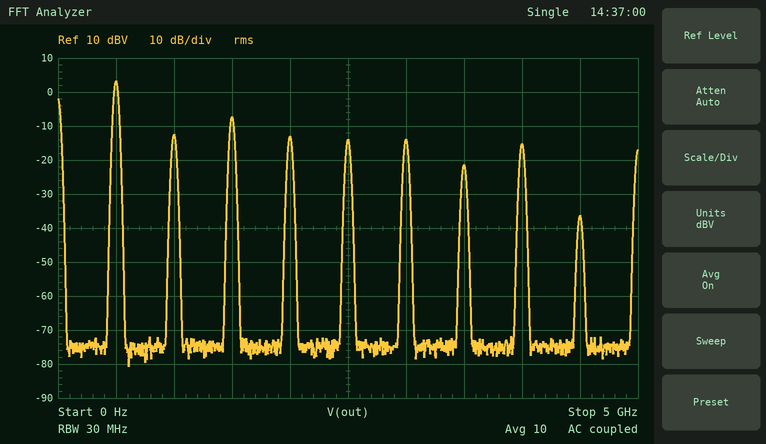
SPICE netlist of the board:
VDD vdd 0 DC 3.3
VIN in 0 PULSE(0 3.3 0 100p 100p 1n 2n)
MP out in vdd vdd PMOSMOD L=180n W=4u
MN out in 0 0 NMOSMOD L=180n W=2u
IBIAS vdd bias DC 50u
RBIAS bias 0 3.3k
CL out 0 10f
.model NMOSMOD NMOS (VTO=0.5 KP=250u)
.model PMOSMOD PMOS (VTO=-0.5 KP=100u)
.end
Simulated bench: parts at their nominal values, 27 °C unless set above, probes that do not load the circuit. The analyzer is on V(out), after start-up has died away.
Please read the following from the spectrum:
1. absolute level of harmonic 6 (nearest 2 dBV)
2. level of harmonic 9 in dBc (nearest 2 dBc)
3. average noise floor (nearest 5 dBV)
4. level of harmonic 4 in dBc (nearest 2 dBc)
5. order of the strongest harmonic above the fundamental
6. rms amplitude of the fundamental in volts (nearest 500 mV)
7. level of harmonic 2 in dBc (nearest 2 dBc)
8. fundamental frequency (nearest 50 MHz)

-14 dBV
-40 dBc
-75 dBV
-16 dBc
3
1.5 V
-16 dBc
500 MHz
